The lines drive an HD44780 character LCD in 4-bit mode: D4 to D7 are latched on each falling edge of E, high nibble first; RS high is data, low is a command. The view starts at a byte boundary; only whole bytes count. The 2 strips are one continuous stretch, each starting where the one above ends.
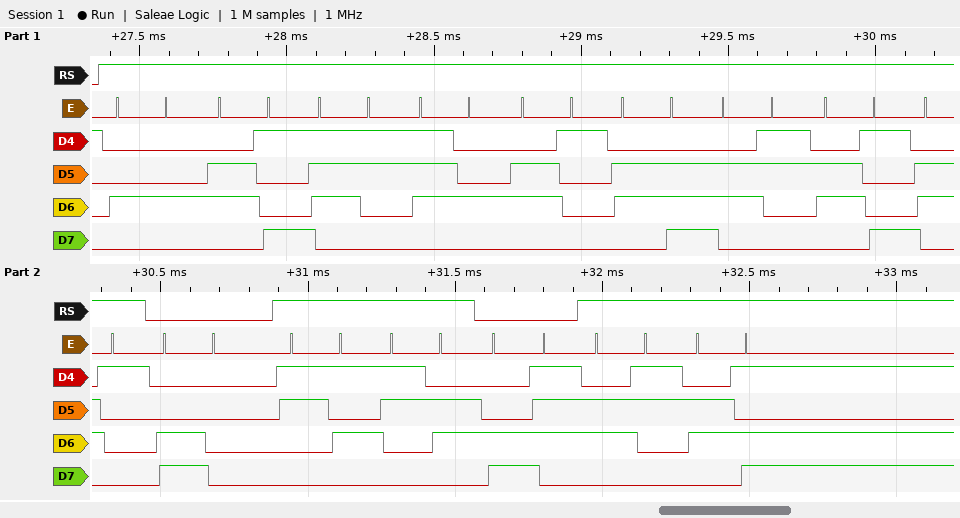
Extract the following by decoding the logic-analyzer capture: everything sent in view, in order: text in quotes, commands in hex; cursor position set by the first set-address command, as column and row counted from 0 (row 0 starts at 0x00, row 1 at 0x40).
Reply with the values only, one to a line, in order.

"Distancia" 0xC0 "56" 0xC7 "cm"
column 0, row 1
